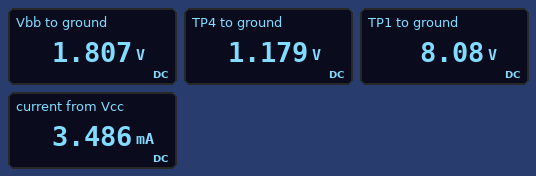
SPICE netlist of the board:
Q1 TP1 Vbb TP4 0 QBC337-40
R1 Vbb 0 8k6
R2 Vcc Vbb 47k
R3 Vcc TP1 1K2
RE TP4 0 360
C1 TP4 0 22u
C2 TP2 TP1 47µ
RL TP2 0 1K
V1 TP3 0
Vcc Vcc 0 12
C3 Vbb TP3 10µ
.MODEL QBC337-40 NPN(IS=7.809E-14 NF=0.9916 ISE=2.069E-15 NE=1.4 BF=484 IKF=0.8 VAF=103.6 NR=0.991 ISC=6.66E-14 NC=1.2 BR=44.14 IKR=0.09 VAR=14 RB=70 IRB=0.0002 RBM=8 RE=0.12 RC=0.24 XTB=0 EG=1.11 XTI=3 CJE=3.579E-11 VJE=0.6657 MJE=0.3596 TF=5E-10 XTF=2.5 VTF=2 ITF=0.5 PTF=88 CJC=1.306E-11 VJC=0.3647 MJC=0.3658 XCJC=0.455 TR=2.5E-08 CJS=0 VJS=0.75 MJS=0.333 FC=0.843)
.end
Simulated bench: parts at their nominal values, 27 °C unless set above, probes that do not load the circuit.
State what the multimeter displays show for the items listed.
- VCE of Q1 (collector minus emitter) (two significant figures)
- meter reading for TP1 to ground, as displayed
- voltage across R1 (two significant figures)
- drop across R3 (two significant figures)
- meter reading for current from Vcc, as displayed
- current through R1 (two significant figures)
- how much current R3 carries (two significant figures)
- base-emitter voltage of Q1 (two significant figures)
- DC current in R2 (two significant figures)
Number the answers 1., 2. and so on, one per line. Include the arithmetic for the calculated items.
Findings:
1. 8.08 V - 1.179 V = 6.9 V
2. 8.08 V
3. 1.807 V = 1.8 V
4. 12 V - 8.08 V = 3.9 V
5. 3.486 mA
6. (1.807 V) / 8.6 kΩ = 210 µA
7. (12 V - 8.08 V) / 1.2 kΩ = 3.3 mA
8. 1.807 V - 1.179 V = 630 mV
9. (12 V - 1.807 V) / 47 kΩ = 220 µA
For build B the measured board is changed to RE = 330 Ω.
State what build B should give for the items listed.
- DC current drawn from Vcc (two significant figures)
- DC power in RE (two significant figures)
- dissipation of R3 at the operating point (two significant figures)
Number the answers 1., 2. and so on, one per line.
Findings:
1. 3.8 mA
2. 4.2 mW
3. 15 mW
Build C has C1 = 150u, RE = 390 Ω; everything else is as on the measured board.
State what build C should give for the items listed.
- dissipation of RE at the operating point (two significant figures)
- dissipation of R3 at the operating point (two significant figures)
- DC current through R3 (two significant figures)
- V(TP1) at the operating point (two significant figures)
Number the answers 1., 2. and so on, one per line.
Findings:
1. 3.6 mW
2. 11 mW
3. 3.0 mA
4. 8.4 V
